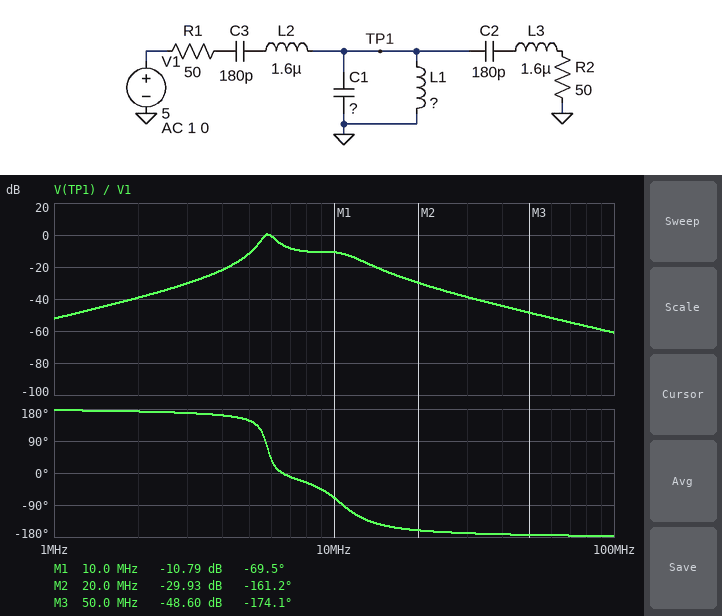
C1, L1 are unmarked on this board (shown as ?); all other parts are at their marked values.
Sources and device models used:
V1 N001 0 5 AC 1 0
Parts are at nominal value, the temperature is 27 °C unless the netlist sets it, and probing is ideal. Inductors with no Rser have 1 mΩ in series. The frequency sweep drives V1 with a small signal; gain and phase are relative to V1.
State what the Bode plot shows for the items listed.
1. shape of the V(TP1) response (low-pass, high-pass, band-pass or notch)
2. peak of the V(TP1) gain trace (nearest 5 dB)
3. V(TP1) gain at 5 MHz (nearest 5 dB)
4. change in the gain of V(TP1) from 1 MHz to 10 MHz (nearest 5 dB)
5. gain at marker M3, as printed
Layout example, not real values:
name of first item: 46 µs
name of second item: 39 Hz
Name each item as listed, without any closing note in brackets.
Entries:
shape of the V(TP1) response: band-pass
peak of the V(TP1) gain trace: 0 dB
V(TP1) gain at 5 MHz: -10 dB
change in the gain of V(TP1) from 1 MHz to 10 MHz: 40 dB
gain at marker M3, as printed: -48.60 dB
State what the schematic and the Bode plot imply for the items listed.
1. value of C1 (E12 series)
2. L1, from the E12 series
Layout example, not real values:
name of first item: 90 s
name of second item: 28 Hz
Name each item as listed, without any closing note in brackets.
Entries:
value of C1: 1.8 nF
L1, from the E12 series: 330 nH
